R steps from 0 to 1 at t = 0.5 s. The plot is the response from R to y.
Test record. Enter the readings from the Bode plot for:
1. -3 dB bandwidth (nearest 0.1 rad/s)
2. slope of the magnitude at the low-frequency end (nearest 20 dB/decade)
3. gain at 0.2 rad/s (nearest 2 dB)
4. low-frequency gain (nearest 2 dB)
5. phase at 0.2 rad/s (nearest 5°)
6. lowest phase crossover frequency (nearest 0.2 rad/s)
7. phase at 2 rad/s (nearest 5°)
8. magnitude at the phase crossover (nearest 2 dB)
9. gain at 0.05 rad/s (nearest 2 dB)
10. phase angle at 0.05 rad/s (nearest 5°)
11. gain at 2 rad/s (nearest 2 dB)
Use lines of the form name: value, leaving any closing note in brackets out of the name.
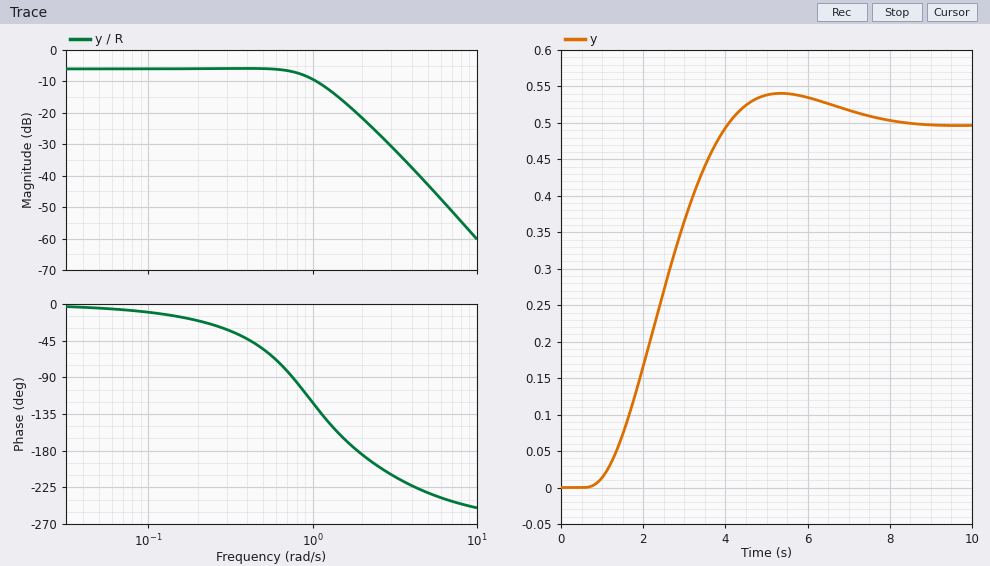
-3 dB bandwidth: 1.0 rad/s
slope of the magnitude at the low-frequency end: 0 dB/decade
gain at 0.2 rad/s: -6 dB
low-frequency gain: -6 dB
phase at 0.2 rad/s: -20°
lowest phase crossover frequency: 1.8 rad/s
phase at 2 rad/s: -185°
magnitude at the phase crossover: -20 dB
gain at 0.05 rad/s: -6 dB
phase angle at 0.05 rad/s: -5°
gain at 2 rad/s: -22 dB
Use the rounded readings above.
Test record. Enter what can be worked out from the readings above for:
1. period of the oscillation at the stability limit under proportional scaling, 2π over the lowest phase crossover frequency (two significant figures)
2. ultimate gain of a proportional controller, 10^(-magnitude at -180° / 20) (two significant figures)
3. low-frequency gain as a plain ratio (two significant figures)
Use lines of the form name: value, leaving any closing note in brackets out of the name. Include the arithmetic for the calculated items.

period of the oscillation at the stability limit under proportional scaling, 2π over the lowest phase crossover frequency: 2π / 1.8 = 3.5 s
ultimate gain of a proportional controller, 10^(-magnitude at -180° / 20): 10^(20 / 20) = 10
low-frequency gain as a plain ratio: 10^(-6 / 20) = 0.50
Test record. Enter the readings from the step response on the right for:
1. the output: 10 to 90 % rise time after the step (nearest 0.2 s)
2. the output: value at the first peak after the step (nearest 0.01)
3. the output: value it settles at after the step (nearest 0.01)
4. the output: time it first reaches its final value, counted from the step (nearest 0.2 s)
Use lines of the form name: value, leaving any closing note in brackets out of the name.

the output: 10 to 90 % rise time after the step: 2.2 s
the output: value at the first peak after the step: 0.54
the output: value it settles at after the step: 0.50
the output: time it first reaches its final value, counted from the step: 3.6 s
